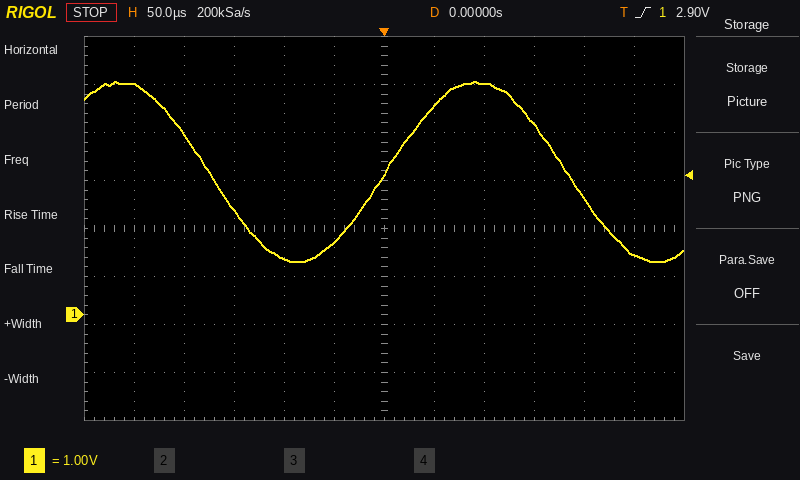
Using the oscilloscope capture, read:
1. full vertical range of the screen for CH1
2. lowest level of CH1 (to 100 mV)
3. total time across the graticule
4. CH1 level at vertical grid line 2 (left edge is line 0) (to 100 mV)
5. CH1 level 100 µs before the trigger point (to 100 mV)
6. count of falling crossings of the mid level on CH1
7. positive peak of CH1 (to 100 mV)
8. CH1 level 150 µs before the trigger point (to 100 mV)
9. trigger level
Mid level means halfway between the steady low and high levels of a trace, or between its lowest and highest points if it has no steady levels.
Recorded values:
8 V
1.1 V
600 µs
3.8 V
1.2 V
2
4.9 V
2.2 V
2.90 V
